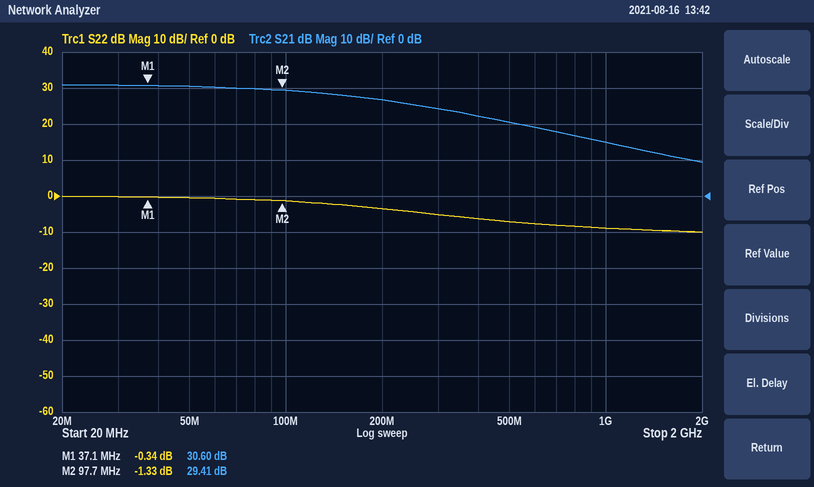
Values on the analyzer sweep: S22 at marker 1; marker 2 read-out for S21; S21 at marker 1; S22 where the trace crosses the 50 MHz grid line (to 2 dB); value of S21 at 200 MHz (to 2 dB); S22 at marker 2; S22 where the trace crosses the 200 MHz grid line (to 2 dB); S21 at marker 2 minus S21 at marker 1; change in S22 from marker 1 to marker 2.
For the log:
-0.34 dB
29.41 dB
30.60 dB
0 dB
26 dB
-1.33 dB
-4 dB
-1.19 dB
-0.99 dB
